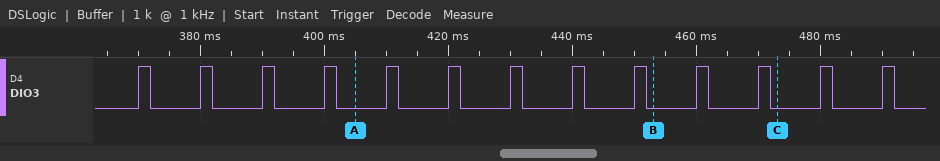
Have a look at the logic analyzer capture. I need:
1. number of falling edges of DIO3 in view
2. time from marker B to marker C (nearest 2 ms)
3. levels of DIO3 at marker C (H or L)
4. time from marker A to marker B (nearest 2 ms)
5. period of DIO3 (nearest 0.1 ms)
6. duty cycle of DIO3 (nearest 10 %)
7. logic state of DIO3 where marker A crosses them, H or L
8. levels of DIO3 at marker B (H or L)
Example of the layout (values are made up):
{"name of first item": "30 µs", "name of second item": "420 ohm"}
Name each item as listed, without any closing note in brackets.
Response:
{"number of falling edges of DIO3 in view": "13", "time from marker B to marker C": "20 ms", "levels of DIO3 at marker C": "DIO3=L", "time from marker A to marker B": "48 ms", "period of DIO3": "10 ms", "duty cycle of DIO3": "20 %", "logic state of DIO3 where marker A crosses them, H or L": "DIO3=L", "levels of DIO3 at marker B": "DIO3=L"}
